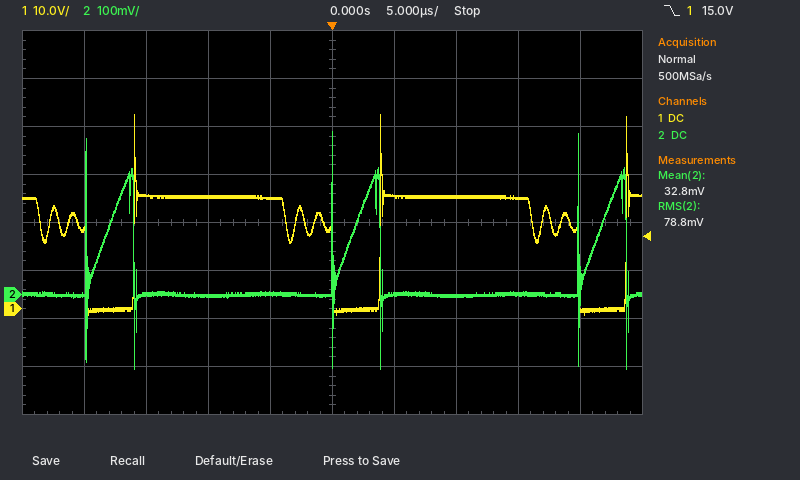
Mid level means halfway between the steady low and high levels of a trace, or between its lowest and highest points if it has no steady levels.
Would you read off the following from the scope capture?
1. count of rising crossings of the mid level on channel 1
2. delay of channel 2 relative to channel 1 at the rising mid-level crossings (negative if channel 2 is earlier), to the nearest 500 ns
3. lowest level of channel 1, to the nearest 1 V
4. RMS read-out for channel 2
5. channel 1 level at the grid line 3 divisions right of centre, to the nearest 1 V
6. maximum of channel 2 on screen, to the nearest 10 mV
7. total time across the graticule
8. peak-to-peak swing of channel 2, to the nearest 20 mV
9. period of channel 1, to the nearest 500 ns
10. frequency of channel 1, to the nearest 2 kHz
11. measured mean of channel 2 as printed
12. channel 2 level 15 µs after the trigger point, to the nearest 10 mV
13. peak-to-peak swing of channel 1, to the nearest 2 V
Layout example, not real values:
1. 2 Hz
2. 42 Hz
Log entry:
1. 3
2. -2.5 µs
3. -1 V
4. 78.8 mV
5. 23 V
6. 340 mV
7. 50 µs
8. 500 mV
9. 20.0 µs
10. 50 kHz
11. 32.8 mV
12. 0 mV
13. 42 V
